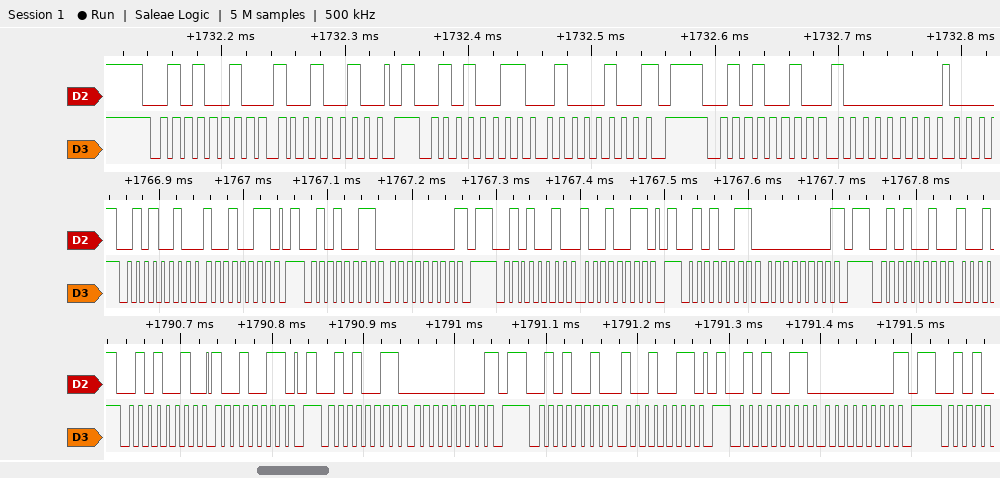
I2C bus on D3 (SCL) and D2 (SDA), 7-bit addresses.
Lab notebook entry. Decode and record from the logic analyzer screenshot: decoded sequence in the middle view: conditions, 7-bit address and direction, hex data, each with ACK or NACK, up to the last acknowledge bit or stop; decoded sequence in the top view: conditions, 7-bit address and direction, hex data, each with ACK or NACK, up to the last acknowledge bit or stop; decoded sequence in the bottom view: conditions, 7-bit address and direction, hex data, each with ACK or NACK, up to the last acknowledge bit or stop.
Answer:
start, address 29 write ACK, 93 ACK, stop, start, address 29 read ACK, 00 NACK, stop, start, address 29 write ACK, 93 ACK, stop, start, address 29 read ACK, 00 NACK, stop, start, address 29 write ACK
start, address 29 write ACK, 92 ACK, stop, start, address 29 read ACK, 44 NACK, stop, start, address 29 write ACK, 80 ACK
start, address 29 write ACK, 93 ACK, stop, start, address 29 read ACK, 00 NACK, stop, start, address 29 write ACK, 93 ACK, stop, start, address 29 read ACK, 00 NACK, stop
